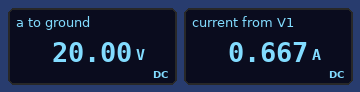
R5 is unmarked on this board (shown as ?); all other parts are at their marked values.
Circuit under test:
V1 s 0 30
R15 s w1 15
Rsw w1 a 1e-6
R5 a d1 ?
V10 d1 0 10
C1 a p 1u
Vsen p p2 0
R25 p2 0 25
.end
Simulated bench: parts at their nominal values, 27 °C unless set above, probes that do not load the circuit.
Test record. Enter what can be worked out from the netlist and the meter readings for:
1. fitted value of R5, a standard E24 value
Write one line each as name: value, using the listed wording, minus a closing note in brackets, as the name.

fitted value of R5, a standard E24 value: 15 Ω
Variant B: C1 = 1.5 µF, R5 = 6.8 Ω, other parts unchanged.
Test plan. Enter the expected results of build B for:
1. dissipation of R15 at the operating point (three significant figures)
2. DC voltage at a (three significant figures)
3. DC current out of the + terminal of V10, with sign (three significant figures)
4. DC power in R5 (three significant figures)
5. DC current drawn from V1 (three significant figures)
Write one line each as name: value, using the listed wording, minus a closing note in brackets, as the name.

dissipation of R15 at the operating point: 12.6 W
DC voltage at a: 16.2 V
DC current out of the + terminal of V10, with sign: -917 mA
DC power in R5: 5.72 W
DC current drawn from V1: 917 mA
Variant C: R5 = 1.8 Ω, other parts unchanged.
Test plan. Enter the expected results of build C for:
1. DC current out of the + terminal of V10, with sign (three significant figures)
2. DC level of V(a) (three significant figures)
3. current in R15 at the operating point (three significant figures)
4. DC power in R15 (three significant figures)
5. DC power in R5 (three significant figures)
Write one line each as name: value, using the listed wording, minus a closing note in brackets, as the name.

DC current out of the + terminal of V10, with sign: -1.19 A
DC level of V(a): 12.1 V
current in R15 at the operating point: 1.19 A
DC power in R15: 21.3 W
DC power in R5: 2.55 W
